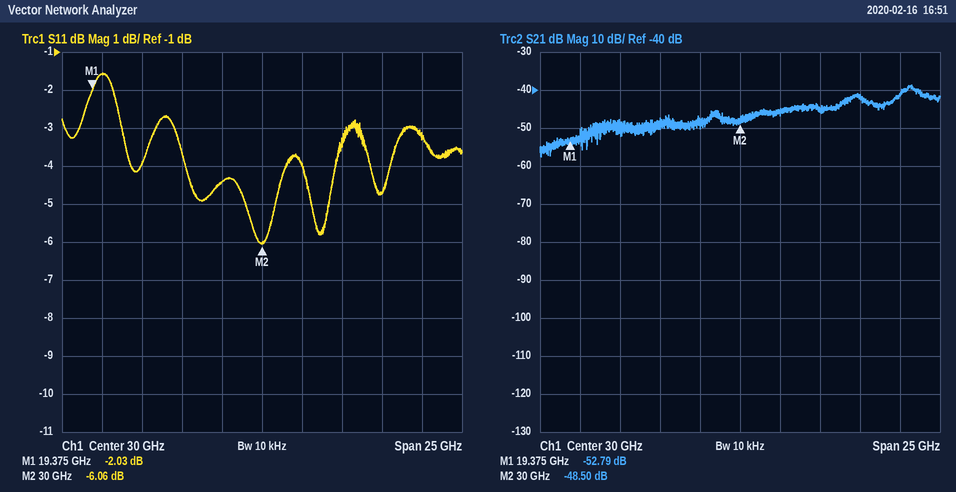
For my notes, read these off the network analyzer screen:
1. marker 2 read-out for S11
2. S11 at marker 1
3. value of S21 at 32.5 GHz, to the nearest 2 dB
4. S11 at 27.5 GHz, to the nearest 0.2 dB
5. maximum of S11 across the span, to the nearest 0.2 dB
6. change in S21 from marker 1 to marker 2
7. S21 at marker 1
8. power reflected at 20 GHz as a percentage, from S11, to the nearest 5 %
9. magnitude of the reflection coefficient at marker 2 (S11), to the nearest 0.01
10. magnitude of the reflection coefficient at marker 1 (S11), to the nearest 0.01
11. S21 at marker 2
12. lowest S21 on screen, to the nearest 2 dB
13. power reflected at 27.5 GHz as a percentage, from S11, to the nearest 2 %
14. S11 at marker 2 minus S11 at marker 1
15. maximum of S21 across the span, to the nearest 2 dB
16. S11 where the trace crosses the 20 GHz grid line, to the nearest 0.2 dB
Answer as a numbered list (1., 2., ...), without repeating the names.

1. -6.06 dB
2. -2.03 dB
3. -46 dB
4. -4.4 dB
5. -1.6 dB
6. 4.29 dB
7. -52.79 dB
8. 70 %
9. 0.50
10. 0.79
11. -48.50 dB
12. -58 dB
13. 36 %
14. -4.03 dB
15. -38 dB
16. -1.6 dB
